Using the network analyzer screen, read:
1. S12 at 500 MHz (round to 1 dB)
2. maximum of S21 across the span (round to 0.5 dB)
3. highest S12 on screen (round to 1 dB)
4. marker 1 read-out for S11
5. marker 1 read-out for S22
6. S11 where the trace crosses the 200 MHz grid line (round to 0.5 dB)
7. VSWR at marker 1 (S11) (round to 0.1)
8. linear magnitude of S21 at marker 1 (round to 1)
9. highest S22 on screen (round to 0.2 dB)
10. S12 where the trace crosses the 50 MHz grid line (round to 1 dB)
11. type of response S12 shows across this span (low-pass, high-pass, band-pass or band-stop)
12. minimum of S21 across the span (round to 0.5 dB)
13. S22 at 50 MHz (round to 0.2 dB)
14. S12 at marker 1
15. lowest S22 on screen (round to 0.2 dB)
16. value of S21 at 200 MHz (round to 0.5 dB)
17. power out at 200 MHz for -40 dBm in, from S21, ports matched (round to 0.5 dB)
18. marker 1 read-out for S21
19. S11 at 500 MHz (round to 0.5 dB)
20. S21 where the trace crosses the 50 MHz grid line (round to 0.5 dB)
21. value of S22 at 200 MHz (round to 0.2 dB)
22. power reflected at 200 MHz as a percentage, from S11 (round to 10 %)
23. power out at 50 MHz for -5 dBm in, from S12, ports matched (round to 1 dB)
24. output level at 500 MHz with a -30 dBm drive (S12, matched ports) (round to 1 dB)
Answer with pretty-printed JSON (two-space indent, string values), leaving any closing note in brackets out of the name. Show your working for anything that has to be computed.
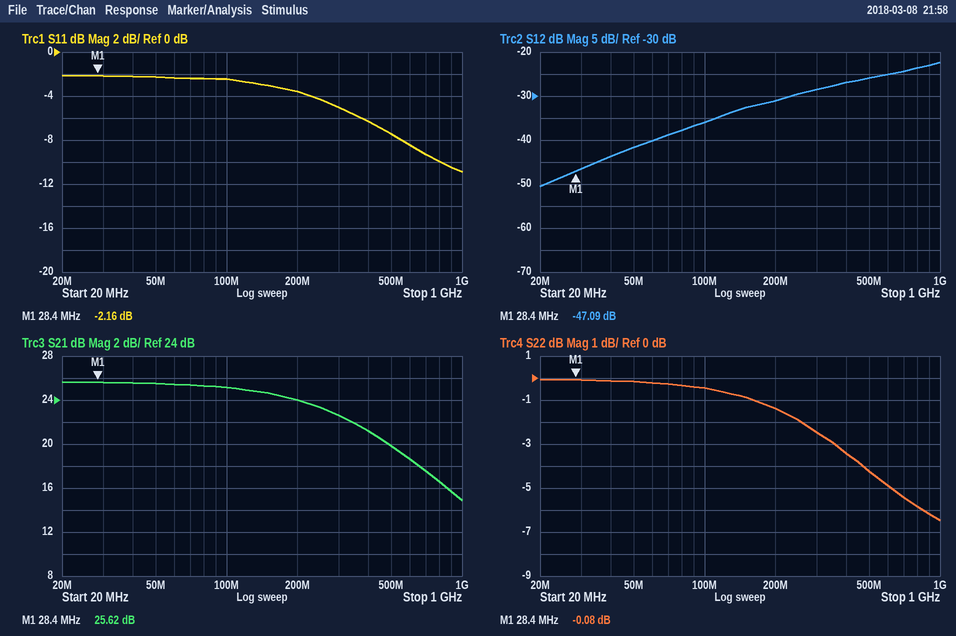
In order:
{
  "S12 at 500 MHz": "-26 dB",
  "maximum of S21 across the span": "25.5 dB",
  "highest S12 on screen": "-22 dB",
  "marker 1 read-out for S11": "-2.16 dB",
  "marker 1 read-out for S22": "-0.08 dB",
  "S11 where the trace crosses the 200 MHz grid line": "-3.5 dB",
  "VSWR at marker 1 (S11)": "(1 + 0.7798)/(1 − 0.7798) ≈ 8.1",
  "linear magnitude of S21 at marker 1": "10^(25.62/20) ≈ 19",
  "highest S22 on screen": "0.0 dB",
  "S12 where the trace crosses the 50 MHz grid line": "-42 dB",
  "type of response S12 shows across this span": "high-pass",
  "minimum of S21 across the span": "15.0 dB",
  "S22 at 50 MHz": "-0.2 dB",
  "S12 at marker 1": "-47.09 dB",
  "lowest S22 on screen": "-6.4 dB",
  "value of S21 at 200 MHz": "24.0 dB",
  "power out at 200 MHz for -40 dBm in, from S21, ports matched": "-40 dBm + (24.0 dB) = -16.0 dBm",
  "marker 1 read-out for S21": "25.62 dB",
  "S11 at 500 MHz": "-7.5 dB",
  "S21 where the trace crosses the 50 MHz grid line": "25.5 dB",
  "value of S22 at 200 MHz": "-1.4 dB",
  "power reflected at 200 MHz as a percentage, from S11": "10^(-3.5/10) ≈ 44.7 %, so 40 % to the nearest 10 %",
  "power out at 50 MHz for -5 dBm in, from S12, ports matched": "-5 dBm + (-42 dB) = -47 dBm",
  "output level at 500 MHz with a -30 dBm drive (S12, matched ports)": "-30 dBm + (-26 dB) = -56 dBm"
}
